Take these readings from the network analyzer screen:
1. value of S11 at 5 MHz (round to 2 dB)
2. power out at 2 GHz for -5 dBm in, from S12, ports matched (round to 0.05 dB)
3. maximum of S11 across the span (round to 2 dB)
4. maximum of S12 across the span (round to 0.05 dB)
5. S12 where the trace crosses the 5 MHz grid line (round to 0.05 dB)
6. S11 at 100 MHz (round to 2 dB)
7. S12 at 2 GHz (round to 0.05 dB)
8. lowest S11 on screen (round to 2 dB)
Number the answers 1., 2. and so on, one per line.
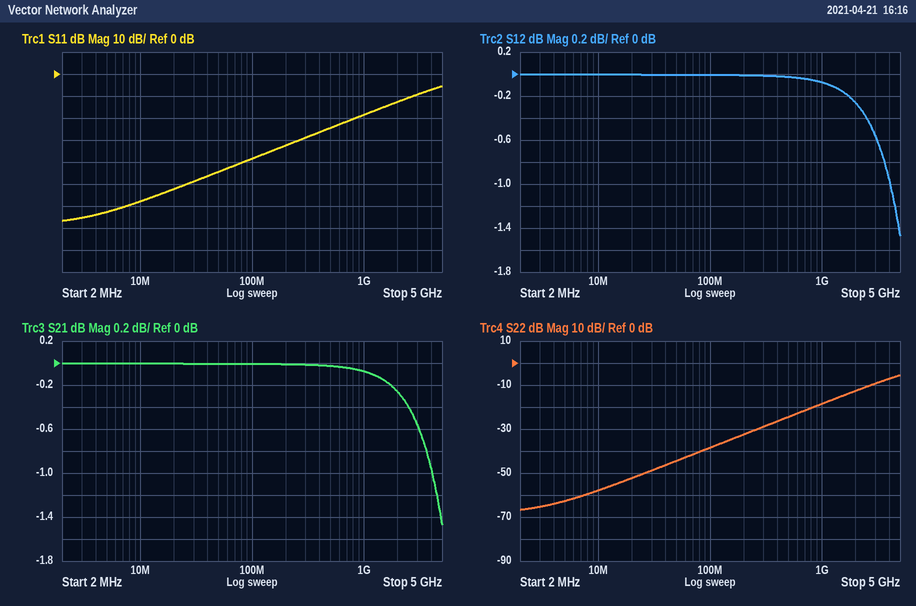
1. -62 dB
2. -5.25 dBm
3. -6 dB
4. 0.00 dB
5. 0.00 dB
6. -38 dB
7. -0.25 dB
8. -66 dB
